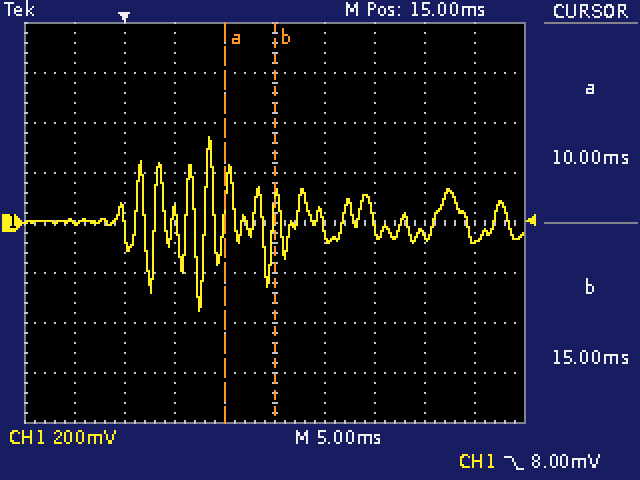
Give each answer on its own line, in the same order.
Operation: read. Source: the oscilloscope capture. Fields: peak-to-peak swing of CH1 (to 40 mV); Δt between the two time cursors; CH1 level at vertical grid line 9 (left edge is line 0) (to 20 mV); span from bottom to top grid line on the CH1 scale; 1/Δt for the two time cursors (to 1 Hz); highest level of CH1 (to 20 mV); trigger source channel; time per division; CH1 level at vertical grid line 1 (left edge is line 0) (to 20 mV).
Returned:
680 mV
5.0 ms
-60 mV
1.6 V
200 Hz
340 mV
CH1
5 ms
0 mV
